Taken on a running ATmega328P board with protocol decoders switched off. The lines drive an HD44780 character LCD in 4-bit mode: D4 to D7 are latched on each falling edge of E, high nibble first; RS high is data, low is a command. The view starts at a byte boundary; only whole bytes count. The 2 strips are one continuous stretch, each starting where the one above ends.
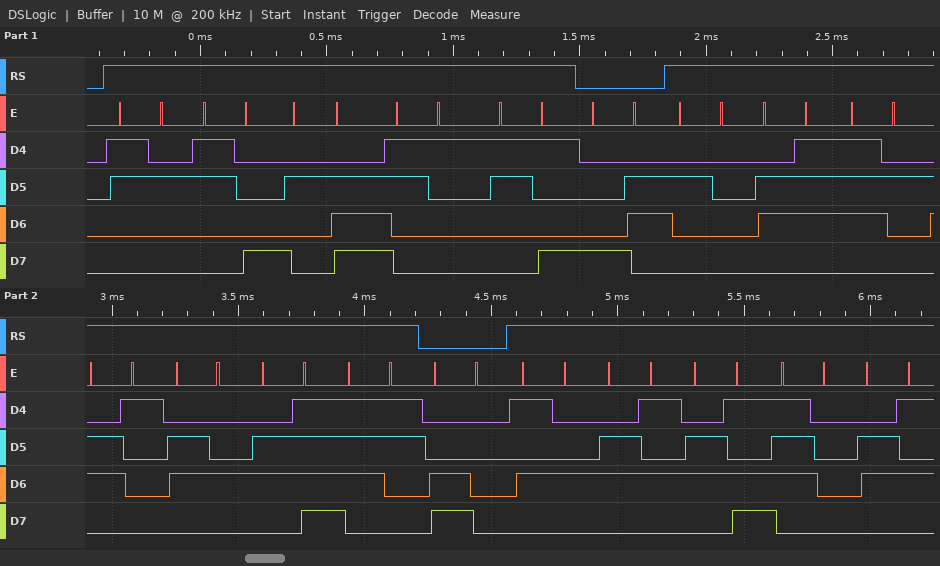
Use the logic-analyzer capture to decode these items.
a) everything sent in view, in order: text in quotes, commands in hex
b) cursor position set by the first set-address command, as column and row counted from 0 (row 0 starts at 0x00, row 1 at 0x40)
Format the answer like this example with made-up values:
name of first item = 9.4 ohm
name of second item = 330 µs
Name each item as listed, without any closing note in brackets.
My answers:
everything sent in view, in order: text in quotes, commands in hex = "28.19" 0x86 " grados" 0xC0 "Tempe"
cursor position set by the first set-address command, as column and row counted from 0 = column 6, row 0
